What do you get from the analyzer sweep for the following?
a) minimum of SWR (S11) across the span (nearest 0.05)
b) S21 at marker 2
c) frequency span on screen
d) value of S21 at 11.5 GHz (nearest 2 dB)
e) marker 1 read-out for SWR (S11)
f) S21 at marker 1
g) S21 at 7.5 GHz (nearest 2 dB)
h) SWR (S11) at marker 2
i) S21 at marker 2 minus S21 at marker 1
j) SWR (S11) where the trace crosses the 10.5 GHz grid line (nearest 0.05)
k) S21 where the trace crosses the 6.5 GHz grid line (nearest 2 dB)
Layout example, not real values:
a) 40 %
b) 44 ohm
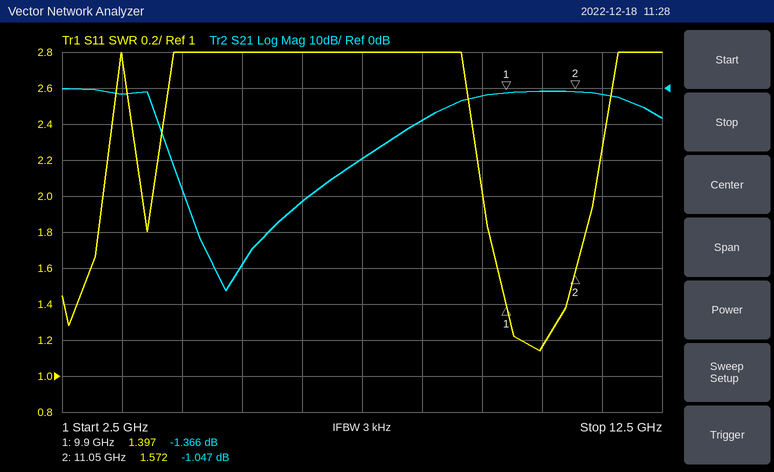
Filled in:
a) 1.15
b) -1.047 dB
c) 10 GHz
d) -2 dB
e) 1.397
f) -1.366 dB
g) -20 dB
h) 1.572
i) 0.319 dB
j) 1.15
k) -32 dB
